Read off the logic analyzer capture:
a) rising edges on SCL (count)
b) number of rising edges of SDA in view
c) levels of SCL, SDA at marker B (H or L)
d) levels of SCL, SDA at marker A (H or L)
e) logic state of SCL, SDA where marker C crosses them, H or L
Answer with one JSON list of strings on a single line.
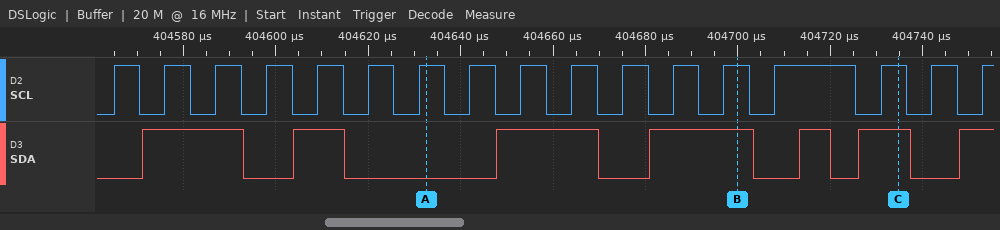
["17", "7", "SCL=H, SDA=H", "SCL=H, SDA=L", "SCL=H, SDA=H"]
